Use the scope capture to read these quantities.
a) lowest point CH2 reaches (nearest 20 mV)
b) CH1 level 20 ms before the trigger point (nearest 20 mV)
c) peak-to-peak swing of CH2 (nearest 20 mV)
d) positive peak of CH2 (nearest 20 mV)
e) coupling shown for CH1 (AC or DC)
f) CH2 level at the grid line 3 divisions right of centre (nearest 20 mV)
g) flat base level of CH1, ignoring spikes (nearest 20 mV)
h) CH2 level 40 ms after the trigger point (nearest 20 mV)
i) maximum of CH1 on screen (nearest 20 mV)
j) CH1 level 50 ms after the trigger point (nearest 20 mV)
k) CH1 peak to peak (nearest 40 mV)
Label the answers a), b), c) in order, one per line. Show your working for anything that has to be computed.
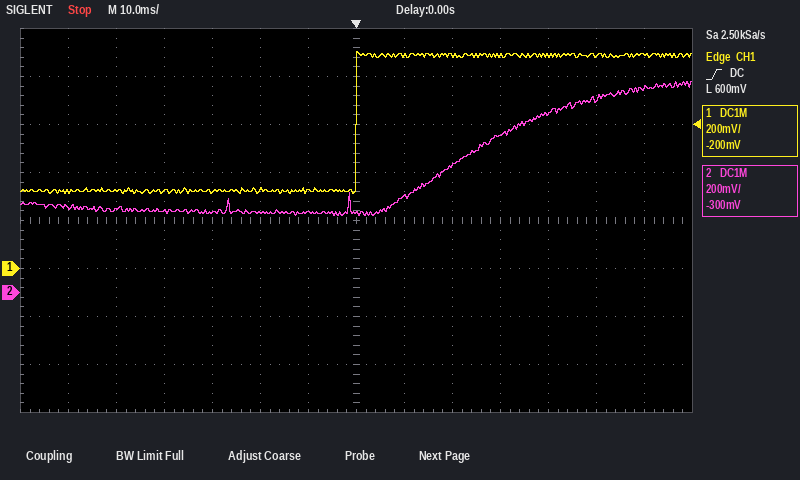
a) 320 mV
b) 320 mV
c) 880 mV − (320 mV) = 560 mV
d) 880 mV
e) DC
f) 660 mV
g) 320 mV
h) 740 mV
i) 900 mV
j) 880 mV
k) 600 mV
